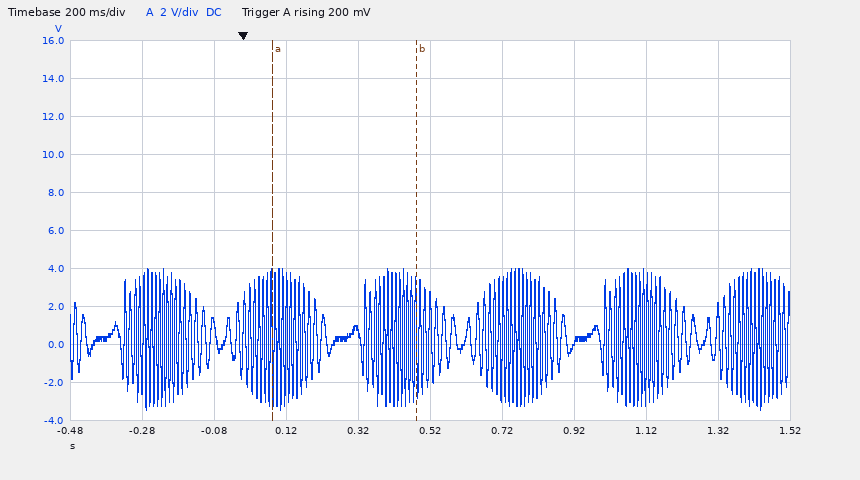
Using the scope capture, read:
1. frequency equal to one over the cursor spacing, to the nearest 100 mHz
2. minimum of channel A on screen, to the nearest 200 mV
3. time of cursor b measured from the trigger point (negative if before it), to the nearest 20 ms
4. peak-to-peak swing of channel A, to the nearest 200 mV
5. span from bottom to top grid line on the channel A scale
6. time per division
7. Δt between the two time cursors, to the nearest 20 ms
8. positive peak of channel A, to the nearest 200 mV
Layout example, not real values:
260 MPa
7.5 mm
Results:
2.5 Hz
-3.4 V
+480 ms
7.4 V
20 V
200 ms
400 ms
4.0 V
